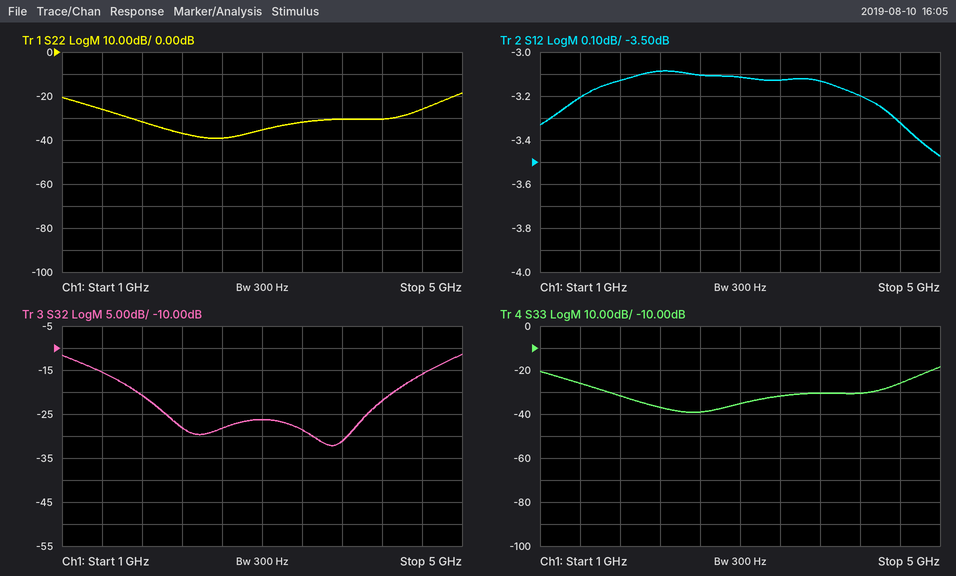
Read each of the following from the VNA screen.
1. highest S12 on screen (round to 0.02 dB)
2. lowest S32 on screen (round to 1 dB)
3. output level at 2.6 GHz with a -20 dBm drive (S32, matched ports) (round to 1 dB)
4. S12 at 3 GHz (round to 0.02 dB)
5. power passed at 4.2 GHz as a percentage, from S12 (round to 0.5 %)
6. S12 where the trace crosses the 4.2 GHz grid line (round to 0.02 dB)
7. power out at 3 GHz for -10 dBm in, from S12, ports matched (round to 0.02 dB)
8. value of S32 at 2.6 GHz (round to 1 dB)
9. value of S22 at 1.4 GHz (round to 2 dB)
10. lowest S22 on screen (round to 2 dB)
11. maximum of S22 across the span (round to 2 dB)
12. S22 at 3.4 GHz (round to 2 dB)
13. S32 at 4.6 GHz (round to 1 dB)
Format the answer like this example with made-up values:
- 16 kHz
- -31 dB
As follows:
- -3.08 dB
- -32 dB
- -48 dBm
- -3.12 dB
- 48.0 %
- -3.20 dB
- -13.12 dBm
- -28 dB
- -26 dB
- -40 dB
- -18 dB
- -32 dB
- -16 dB
